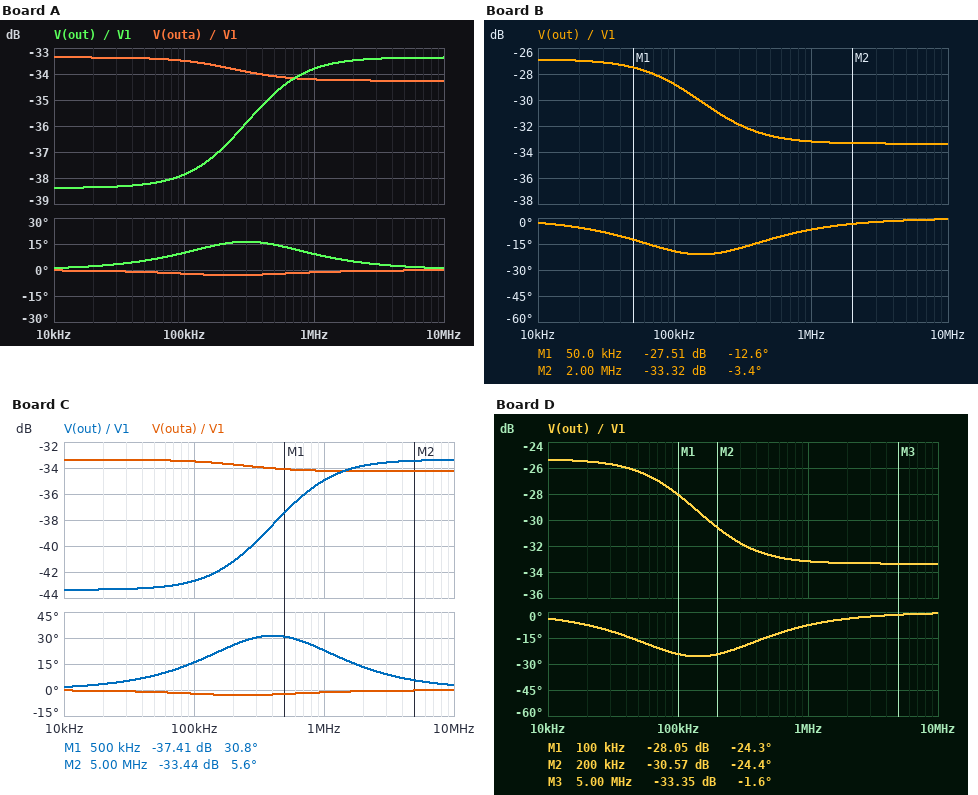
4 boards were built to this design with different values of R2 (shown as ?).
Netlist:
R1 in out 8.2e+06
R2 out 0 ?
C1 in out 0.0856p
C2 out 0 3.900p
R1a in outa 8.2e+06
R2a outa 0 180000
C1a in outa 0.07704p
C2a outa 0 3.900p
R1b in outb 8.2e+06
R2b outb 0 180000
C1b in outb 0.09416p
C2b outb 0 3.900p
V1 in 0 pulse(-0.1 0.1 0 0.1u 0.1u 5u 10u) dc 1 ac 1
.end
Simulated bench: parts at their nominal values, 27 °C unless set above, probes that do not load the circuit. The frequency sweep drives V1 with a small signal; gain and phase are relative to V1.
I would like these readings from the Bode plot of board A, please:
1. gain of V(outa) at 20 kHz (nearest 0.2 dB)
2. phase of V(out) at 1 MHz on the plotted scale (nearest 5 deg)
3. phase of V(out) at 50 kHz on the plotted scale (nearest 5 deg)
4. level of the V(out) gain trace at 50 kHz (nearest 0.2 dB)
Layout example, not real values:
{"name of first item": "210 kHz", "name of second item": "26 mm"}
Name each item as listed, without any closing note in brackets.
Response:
{"gain of V(outa) at 20 kHz": "-33.4 dB", "phase of V(out) at 1 MHz on the plotted scale": "10 deg", "phase of V(out) at 50 kHz on the plotted scale": "5 deg", "level of the V(out) gain trace at 50 kHz": "-38.2 dB"}
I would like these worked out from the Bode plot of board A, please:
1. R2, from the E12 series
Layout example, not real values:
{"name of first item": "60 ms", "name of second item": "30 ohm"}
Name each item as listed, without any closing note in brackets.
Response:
{"R2, from the E12 series": "100 kΩ"}
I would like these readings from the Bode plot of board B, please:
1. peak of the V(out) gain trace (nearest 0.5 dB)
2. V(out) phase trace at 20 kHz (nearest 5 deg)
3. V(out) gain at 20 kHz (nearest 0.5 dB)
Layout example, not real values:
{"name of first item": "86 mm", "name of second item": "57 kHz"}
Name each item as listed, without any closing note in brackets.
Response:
{"peak of the V(out) gain trace": "-27.0 dB", "V(out) phase trace at 20 kHz": "-5 deg", "V(out) gain at 20 kHz": "-27.0 dB"}
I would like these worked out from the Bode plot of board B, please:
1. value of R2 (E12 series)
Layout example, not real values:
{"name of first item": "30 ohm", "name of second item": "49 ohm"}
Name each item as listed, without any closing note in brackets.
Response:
{"value of R2": "390 kΩ"}
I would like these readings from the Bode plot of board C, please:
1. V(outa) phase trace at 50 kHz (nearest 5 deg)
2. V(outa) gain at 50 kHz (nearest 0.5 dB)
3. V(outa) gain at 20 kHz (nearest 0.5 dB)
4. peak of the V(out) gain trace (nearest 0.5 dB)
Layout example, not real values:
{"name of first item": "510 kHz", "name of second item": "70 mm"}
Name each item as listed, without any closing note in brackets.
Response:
{"V(outa) phase trace at 50 kHz": "0 deg", "V(outa) gain at 50 kHz": "-33.5 dB", "V(outa) gain at 20 kHz": "-33.5 dB", "peak of the V(out) gain trace": "-33.5 dB"}
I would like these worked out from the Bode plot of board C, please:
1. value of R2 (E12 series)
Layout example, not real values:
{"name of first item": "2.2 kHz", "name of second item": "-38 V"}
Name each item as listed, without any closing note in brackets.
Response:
{"value of R2": "56 kΩ"}
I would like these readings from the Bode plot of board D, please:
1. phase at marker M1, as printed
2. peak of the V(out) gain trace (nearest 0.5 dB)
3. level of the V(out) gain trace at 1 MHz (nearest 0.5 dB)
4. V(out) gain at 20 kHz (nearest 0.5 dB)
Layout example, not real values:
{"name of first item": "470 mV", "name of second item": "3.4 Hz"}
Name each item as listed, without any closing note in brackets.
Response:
{"phase at marker M1, as printed": "-24.3 deg", "peak of the V(out) gain trace": "-25.5 dB", "level of the V(out) gain trace at 1 MHz": "-33.0 dB", "V(out) gain at 20 kHz": "-25.5 dB"}
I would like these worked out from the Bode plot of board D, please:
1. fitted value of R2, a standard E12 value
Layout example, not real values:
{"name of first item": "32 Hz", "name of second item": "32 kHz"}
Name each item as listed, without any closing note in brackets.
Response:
{"fitted value of R2, a standard E12 value": "470 kΩ"}
